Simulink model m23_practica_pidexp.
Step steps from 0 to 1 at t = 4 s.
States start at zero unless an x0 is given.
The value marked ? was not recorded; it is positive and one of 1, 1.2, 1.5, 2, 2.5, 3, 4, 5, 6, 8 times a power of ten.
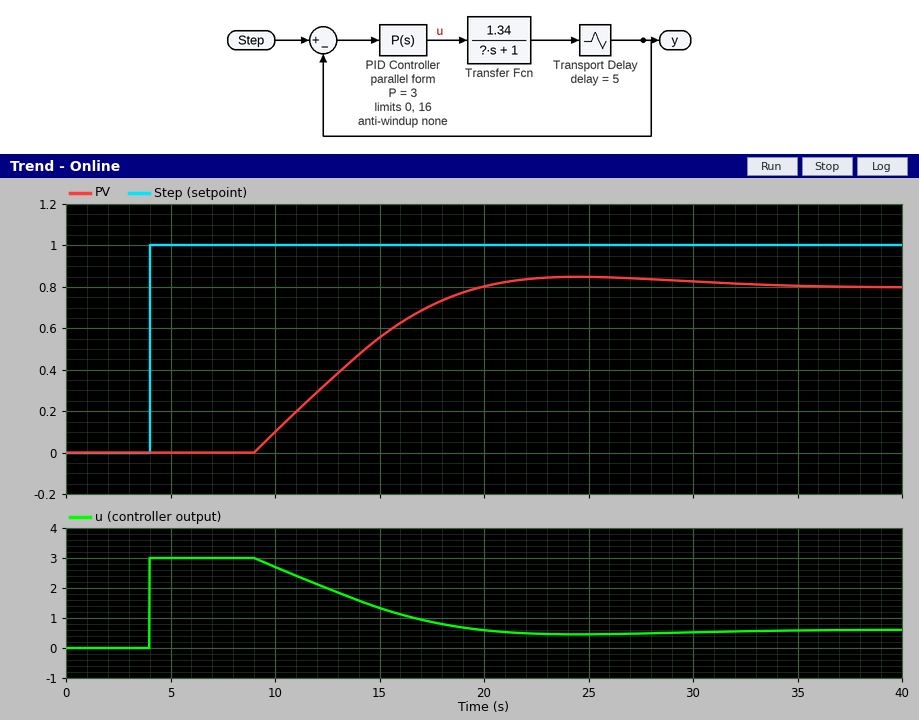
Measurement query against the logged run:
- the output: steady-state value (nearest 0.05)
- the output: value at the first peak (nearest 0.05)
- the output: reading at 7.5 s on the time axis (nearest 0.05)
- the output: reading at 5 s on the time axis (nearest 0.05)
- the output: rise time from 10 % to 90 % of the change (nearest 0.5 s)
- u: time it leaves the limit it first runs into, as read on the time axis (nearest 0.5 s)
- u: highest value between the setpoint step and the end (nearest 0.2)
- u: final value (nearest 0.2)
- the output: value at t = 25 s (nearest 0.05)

0.80
0.85
0.00
0.00
8.0 s
9.0 s
3.0
0.6
0.85
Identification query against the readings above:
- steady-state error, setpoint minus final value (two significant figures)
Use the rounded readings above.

0.20
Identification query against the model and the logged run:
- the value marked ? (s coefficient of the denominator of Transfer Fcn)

40
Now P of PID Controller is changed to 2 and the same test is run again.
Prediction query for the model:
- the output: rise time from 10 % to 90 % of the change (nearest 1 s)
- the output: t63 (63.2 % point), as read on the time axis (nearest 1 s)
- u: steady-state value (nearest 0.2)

14 s
17 s
0.6
